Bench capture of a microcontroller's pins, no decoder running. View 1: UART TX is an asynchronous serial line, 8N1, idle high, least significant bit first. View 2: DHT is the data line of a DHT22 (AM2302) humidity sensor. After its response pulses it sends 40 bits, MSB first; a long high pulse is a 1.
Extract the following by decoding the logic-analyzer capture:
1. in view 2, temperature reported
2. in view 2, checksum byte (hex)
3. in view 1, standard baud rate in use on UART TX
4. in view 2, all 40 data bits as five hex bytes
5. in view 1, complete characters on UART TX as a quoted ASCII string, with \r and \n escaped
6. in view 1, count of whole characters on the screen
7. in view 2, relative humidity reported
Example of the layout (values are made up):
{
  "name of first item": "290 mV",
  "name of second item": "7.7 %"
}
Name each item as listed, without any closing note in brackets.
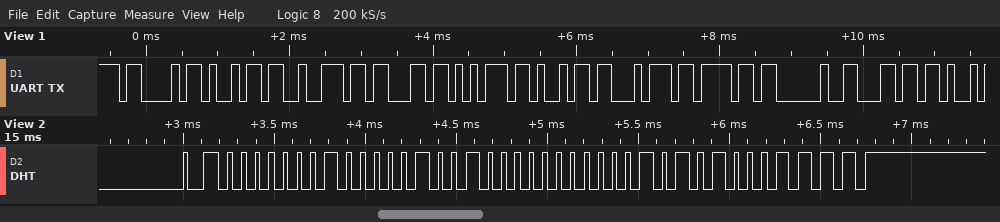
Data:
{
  "in view 2, temperature reported": "-1.0 °C",
  "in view 2, checksum byte": "0x8F",
  "in view 1, standard baud rate in use on UART TX": "9600 baud",
  "in view 2, all 40 data bits as five hex bytes": "01 04 80 0A 8F",
  "in view 1, complete characters on UART TX as a quoted ASCII string, with \\r and \\n escaped": "\"Circuito l\"",
  "in view 1, count of whole characters on the screen": "10",
  "in view 2, relative humidity reported": "26.0 %"
}
